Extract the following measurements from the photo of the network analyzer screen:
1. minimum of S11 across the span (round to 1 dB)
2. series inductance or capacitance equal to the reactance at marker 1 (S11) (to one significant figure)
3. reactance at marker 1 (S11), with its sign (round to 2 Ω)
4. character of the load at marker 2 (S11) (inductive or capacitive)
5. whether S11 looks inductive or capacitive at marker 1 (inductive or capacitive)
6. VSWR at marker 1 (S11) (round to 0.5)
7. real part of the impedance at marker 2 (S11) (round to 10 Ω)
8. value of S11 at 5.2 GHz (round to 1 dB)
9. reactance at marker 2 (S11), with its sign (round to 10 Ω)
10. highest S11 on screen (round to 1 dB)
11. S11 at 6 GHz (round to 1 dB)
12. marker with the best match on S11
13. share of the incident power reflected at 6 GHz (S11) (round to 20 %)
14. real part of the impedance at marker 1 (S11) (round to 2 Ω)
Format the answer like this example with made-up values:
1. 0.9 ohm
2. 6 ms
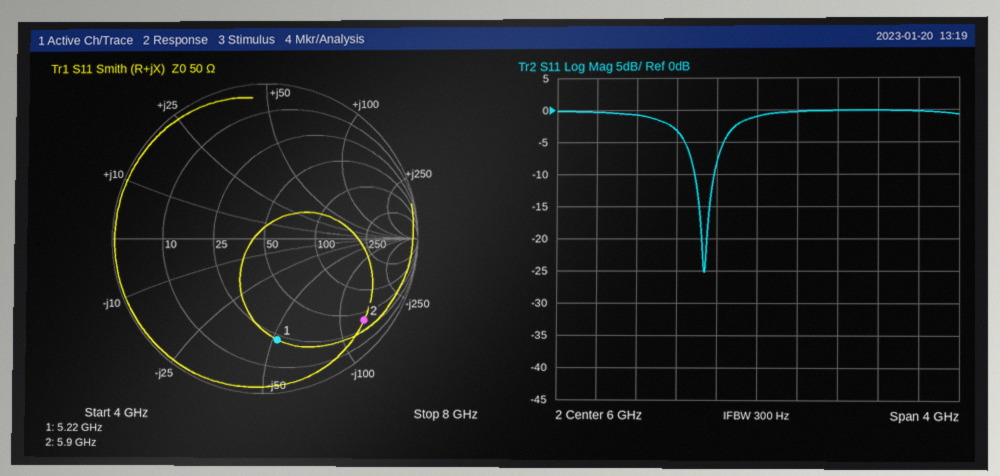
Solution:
1. -25 dB
2. 600 fF
3. -52 Ω
4. capacitive
5. capacitive
6. 5.0
7. 40 Ω
8. -3 dB
9. -130 Ω
10. 0 dB
11. -1 dB
12. marker 1
13. 80 %
14. 22 Ω
